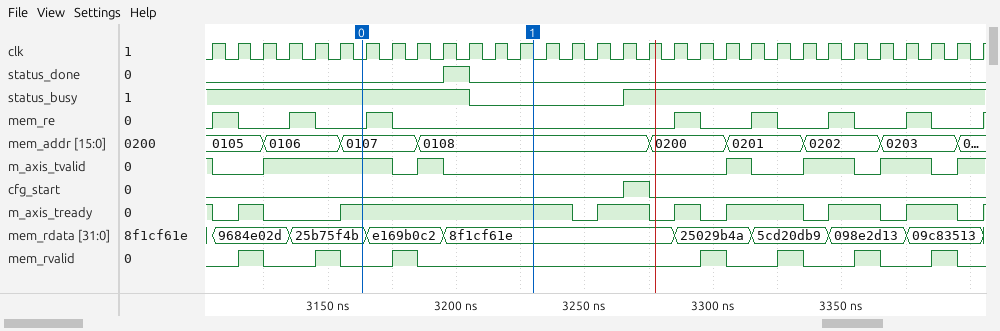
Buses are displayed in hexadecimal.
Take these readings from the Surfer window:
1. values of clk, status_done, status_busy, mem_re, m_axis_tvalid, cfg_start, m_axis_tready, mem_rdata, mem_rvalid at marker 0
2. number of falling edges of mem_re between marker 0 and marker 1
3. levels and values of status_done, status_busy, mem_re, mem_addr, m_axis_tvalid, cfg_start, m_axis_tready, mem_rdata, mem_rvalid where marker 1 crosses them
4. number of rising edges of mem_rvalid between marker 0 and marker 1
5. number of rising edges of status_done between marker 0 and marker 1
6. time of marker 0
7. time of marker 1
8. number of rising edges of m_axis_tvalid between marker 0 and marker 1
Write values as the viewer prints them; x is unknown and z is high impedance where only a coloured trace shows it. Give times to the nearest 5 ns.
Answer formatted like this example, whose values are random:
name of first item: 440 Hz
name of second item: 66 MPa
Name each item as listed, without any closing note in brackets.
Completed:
values of clk, status_done, status_busy, mem_re, m_axis_tvalid, cfg_start, m_axis_tready, mem_rdata, mem_rvalid at marker 0: clk=0, status_done=0, status_busy=1, mem_re=0, m_axis_tvalid=1, cfg_start=0, m_axis_tready=1, mem_rdata=25b75f4b, mem_rvalid=0
number of falling edges of mem_re between marker 0 and marker 1: 1
levels and values of status_done, status_busy, mem_re, mem_addr, m_axis_tvalid, cfg_start, m_axis_tready, mem_rdata, mem_rvalid where marker 1 crosses them: status_done=0, status_busy=0, mem_re=0, mem_addr=0108, m_axis_tvalid=0, cfg_start=0, m_axis_tready=1, mem_rdata=8f1cf61e, mem_rvalid=0
number of rising edges of mem_rvalid between marker 0 and marker 1: 1
number of rising edges of status_done between marker 0 and marker 1: 1
time of marker 0: 3165 ns
time of marker 1: 3230 ns
number of rising edges of m_axis_tvalid between marker 0 and marker 1: 1
